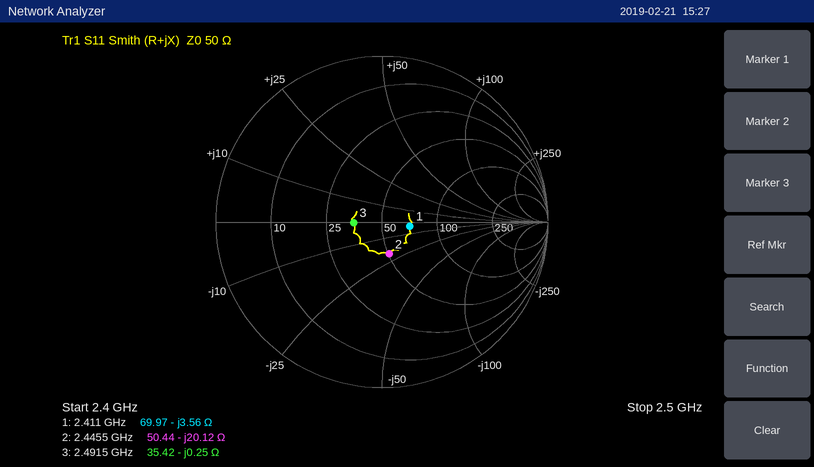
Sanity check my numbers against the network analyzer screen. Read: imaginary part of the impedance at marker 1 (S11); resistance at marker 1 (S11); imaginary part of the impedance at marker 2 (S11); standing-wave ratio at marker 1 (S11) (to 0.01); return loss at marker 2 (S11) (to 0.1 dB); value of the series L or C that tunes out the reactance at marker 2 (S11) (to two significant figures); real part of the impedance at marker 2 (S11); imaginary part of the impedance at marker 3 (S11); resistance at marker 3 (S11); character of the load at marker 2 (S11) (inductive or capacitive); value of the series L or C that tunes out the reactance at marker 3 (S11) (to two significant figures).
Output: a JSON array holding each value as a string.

["-3.56 Ω", "69.97 Ω", "-20.12 Ω", "1.41", "14.1 dB", "1.3 nH", "50.44 Ω", "-0.25 Ω", "35.42 Ω", "capacitive", "16 pH"]
